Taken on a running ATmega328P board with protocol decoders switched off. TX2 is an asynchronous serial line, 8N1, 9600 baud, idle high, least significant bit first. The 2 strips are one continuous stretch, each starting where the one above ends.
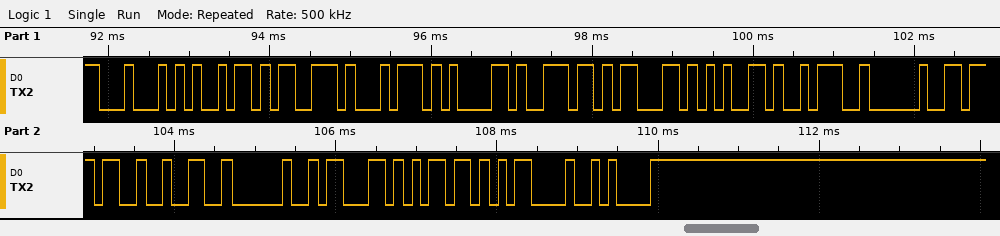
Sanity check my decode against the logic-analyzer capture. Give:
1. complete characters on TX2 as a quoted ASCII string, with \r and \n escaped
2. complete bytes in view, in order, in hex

"Distance: 72 cm\r\n"
0x44 0x69 0x73 0x74 0x61 0x6E 0x63 0x65 0x3A 0x20 0x37 0x32 0x20 0x63 0x6D 0x0D 0x0A
